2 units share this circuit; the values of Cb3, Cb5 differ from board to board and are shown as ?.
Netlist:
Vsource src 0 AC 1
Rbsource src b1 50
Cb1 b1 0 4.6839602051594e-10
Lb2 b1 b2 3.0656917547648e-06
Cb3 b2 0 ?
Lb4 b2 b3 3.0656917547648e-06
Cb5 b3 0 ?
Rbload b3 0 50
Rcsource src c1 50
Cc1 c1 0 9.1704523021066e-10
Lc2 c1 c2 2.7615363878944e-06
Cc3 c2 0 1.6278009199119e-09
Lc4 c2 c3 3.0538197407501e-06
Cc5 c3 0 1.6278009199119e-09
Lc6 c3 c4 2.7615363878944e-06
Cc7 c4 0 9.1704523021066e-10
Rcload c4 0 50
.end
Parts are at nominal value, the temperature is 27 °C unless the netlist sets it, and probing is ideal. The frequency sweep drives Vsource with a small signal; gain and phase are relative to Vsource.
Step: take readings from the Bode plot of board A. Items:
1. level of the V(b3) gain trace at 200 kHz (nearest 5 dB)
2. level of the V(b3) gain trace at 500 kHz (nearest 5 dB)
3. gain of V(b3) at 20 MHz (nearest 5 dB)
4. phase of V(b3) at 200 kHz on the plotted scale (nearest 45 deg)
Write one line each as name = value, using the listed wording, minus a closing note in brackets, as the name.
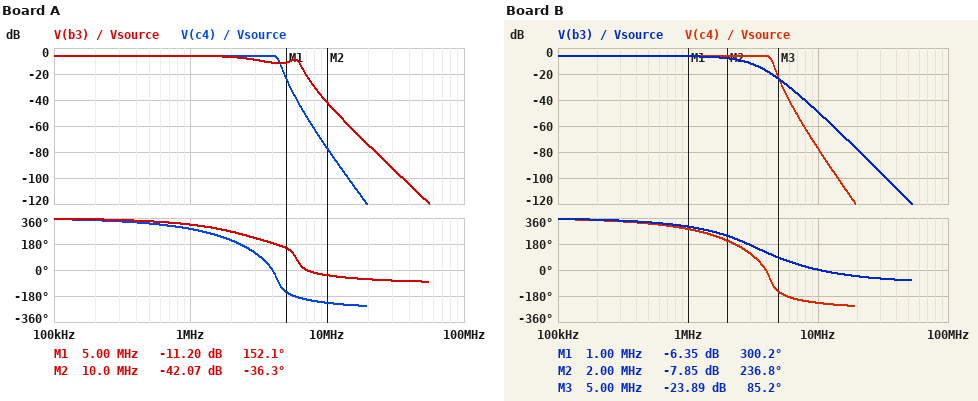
level of the V(b3) gain trace at 200 kHz = -5 dB
level of the V(b3) gain trace at 500 kHz = -5 dB
gain of V(b3) at 20 MHz = -75 dB
phase of V(b3) at 200 kHz on the plotted scale = 360 deg
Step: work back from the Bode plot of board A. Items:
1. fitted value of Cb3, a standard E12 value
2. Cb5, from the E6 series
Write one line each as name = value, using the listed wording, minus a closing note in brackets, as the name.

fitted value of Cb3, a standard E12 value = 560 pF
Cb5, from the E6 series = 1.5 nF
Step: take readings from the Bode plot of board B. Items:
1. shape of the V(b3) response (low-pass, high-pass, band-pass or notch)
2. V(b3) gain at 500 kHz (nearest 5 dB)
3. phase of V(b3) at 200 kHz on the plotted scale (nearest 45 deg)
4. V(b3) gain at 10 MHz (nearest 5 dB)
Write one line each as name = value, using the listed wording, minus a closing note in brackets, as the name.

shape of the V(b3) response = low-pass
V(b3) gain at 500 kHz = -5 dB
phase of V(b3) at 200 kHz on the plotted scale = 360 deg
V(b3) gain at 10 MHz = -50 dB
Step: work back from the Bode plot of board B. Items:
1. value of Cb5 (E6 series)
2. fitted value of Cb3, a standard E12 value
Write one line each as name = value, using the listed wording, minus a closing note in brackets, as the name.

value of Cb5 = 330 pF
fitted value of Cb3, a standard E12 value = 3.3 nF
